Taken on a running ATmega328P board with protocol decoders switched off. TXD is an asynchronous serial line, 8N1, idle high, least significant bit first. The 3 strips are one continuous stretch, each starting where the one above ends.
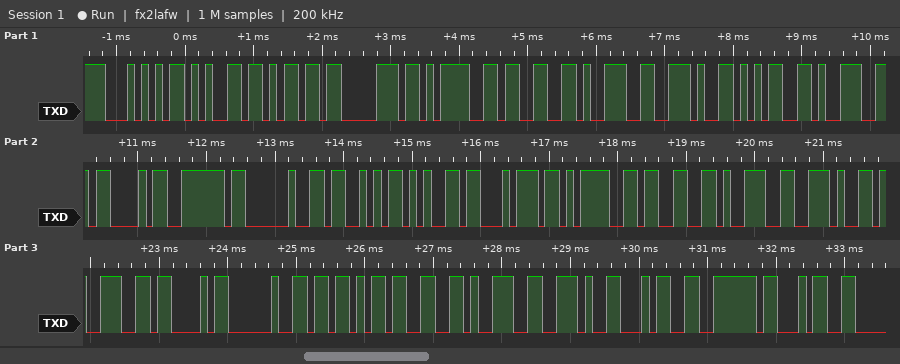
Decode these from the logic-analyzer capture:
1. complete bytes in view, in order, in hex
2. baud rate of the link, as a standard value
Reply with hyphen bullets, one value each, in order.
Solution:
- 54 65 6D 70 3D 33 39 2E 35 39 43 7E 20 53 65 74 3D 33 39 2E 39 43 20 5B 33 39 2E 34 7E 34
- 9600 baud
